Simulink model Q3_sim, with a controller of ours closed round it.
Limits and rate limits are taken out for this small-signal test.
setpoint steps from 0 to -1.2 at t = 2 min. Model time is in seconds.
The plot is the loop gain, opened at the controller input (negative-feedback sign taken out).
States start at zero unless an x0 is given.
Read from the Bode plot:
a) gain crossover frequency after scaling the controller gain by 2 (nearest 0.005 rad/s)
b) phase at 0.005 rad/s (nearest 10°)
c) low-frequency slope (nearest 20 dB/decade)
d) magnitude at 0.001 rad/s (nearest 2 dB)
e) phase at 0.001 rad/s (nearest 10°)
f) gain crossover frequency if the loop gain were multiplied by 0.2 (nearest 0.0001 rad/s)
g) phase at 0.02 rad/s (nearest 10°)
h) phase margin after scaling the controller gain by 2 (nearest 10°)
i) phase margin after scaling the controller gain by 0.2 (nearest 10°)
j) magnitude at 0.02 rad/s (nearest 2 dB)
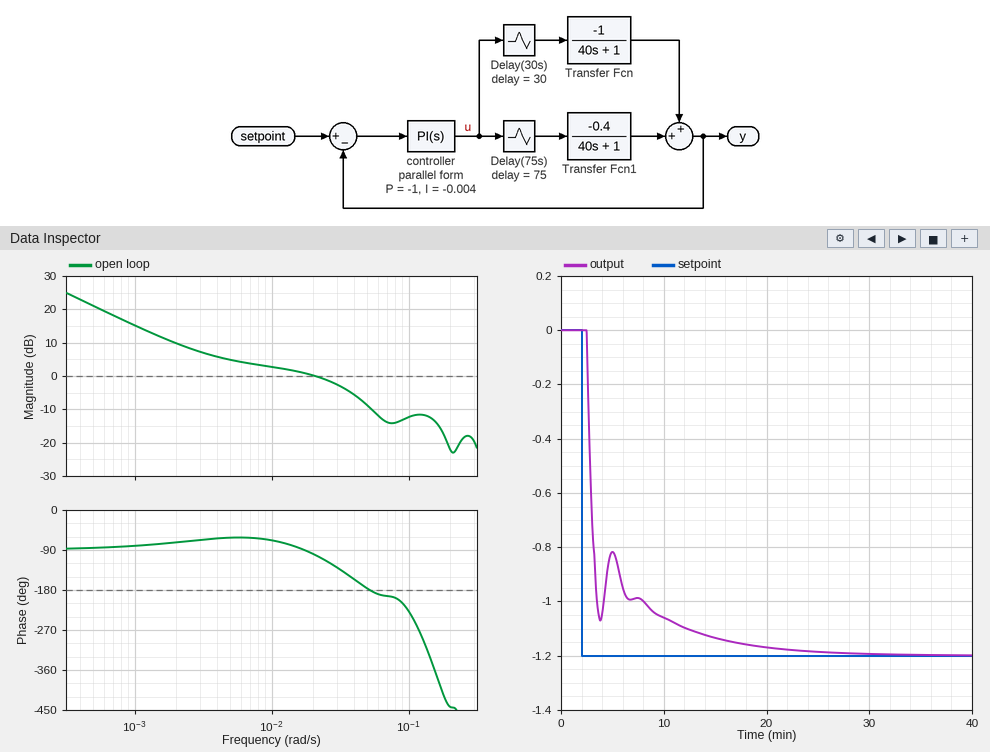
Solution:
0.040 rad/s
-60°
-20 dB/decade
16 dB
-80°
0.0012 rad/s
-100°
20°
100°
0 dB
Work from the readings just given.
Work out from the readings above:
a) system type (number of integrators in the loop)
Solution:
1
